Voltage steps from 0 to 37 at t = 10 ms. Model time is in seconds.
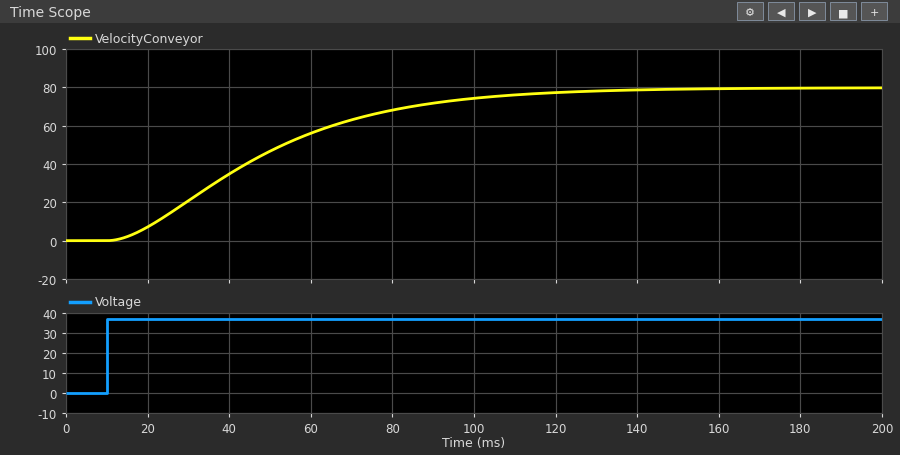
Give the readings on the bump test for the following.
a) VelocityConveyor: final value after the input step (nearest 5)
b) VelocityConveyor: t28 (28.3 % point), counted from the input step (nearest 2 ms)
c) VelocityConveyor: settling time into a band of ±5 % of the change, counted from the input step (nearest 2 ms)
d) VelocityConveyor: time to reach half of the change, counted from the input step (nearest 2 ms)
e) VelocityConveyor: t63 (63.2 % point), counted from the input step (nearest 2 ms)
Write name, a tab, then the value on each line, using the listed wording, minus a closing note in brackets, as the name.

VelocityConveyor: final value after the input step	80
VelocityConveyor: t28 (28.3 % point), counted from the input step	22 ms
VelocityConveyor: settling time into a band of ±5 % of the change, counted from the input step	98 ms
VelocityConveyor: time to reach half of the change, counted from the input step	34 ms
VelocityConveyor: t63 (63.2 % point), counted from the input step	44 ms
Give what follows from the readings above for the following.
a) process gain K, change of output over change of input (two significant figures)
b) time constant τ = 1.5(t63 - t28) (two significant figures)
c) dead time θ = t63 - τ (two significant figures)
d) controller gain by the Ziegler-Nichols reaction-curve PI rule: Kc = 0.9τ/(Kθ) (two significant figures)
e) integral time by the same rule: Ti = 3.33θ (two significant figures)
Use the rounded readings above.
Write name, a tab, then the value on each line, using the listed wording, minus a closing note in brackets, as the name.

process gain K, change of output over change of input	2.2
time constant τ = 1.5(t63 - t28)	33 ms
dead time θ = t63 - τ	11 ms
controller gain by the Ziegler-Nichols reaction-curve PI rule: Kc = 0.9τ/(Kθ)	1.2
integral time by the same rule: Ti = 3.33θ	37 ms
